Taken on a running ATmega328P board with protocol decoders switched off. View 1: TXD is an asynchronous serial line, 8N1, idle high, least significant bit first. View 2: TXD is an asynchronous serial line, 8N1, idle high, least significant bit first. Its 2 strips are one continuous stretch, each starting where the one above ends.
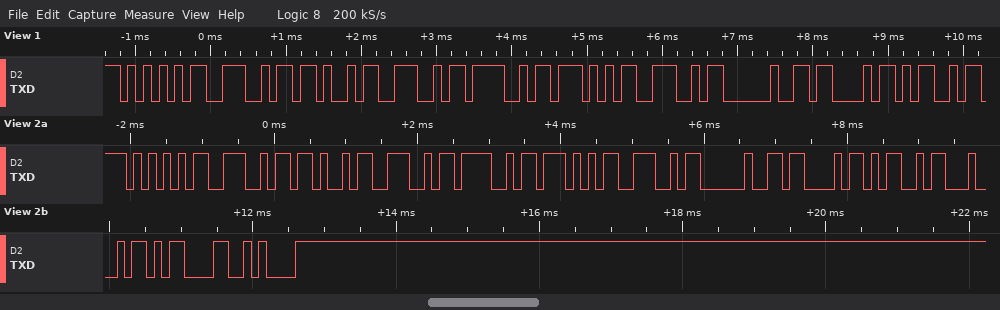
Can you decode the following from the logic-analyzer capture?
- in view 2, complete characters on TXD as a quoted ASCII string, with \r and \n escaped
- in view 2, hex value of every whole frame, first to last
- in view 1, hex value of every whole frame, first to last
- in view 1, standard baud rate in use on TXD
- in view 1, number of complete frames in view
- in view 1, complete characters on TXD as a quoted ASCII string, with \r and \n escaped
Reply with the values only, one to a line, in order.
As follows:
"UNKNOWN CMD\r\n"
0x55 0x4E 0x4B 0x4E 0x4F 0x57 0x4E 0x20 0x43 0x4D 0x44 0x0D 0x0A
0x55 0x4E 0x4B 0x4E 0x4F 0x57 0x4E 0x20 0x43 0x4D
9600 baud
10
"UNKNOWN CM"
